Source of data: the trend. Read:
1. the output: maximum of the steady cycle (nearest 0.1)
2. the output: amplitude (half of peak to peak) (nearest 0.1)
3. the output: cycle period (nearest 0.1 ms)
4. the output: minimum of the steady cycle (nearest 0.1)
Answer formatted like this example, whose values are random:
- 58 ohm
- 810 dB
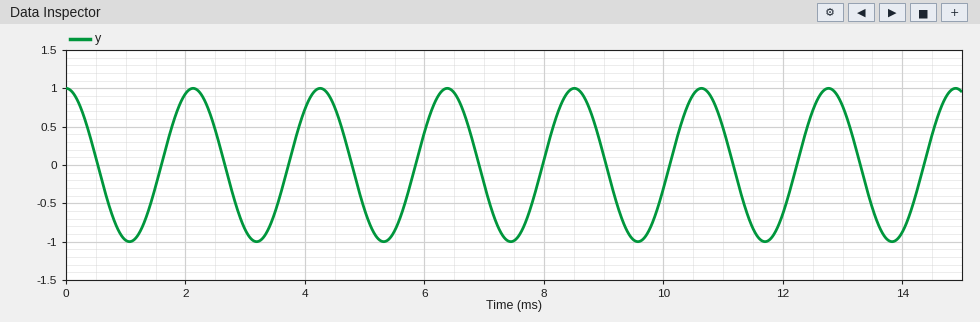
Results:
- 1.0
- 1.0
- 2.1 ms
- -1.0
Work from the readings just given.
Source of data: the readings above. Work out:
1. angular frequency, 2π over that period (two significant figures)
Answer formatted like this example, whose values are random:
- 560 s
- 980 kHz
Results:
- 3.0 rad/ms
